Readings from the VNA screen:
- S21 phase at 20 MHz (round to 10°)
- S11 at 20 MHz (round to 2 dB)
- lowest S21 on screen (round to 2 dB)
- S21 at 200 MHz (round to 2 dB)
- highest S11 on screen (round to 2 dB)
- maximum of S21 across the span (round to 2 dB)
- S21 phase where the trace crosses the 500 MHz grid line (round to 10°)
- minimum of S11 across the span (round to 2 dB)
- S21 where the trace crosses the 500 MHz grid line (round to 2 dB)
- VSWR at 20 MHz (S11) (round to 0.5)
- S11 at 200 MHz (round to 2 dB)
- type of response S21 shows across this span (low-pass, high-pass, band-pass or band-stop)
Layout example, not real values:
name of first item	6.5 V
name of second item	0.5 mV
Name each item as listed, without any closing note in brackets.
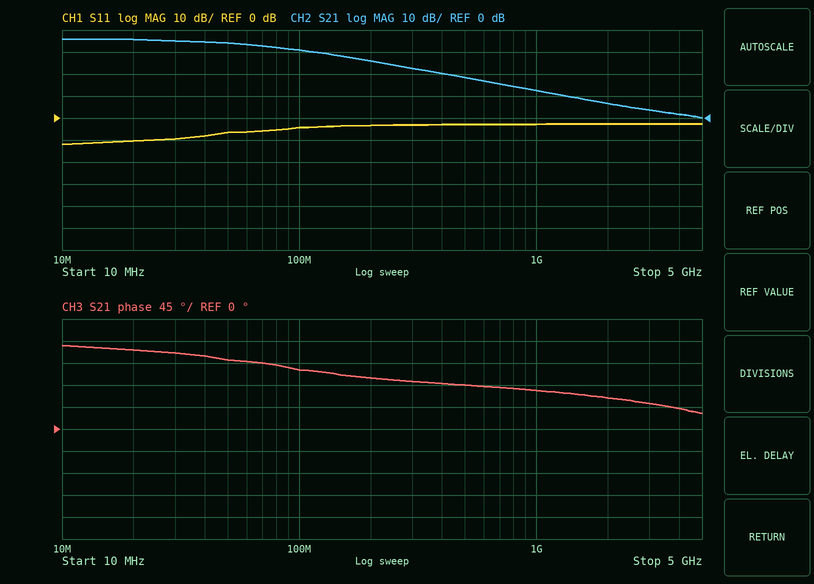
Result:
S21 phase at 20 MHz	160°
S11 at 20 MHz	-10 dB
lowest S21 on screen	0 dB
S21 at 200 MHz	26 dB
highest S11 on screen	-2 dB
maximum of S21 across the span	36 dB
S21 phase where the trace crosses the 500 MHz grid line	90°
minimum of S11 across the span	-12 dB
S21 where the trace crosses the 500 MHz grid line	18 dB
VSWR at 20 MHz (S11)	2.0
S11 at 200 MHz	-4 dB
type of response S21 shows across this span	low-pass
